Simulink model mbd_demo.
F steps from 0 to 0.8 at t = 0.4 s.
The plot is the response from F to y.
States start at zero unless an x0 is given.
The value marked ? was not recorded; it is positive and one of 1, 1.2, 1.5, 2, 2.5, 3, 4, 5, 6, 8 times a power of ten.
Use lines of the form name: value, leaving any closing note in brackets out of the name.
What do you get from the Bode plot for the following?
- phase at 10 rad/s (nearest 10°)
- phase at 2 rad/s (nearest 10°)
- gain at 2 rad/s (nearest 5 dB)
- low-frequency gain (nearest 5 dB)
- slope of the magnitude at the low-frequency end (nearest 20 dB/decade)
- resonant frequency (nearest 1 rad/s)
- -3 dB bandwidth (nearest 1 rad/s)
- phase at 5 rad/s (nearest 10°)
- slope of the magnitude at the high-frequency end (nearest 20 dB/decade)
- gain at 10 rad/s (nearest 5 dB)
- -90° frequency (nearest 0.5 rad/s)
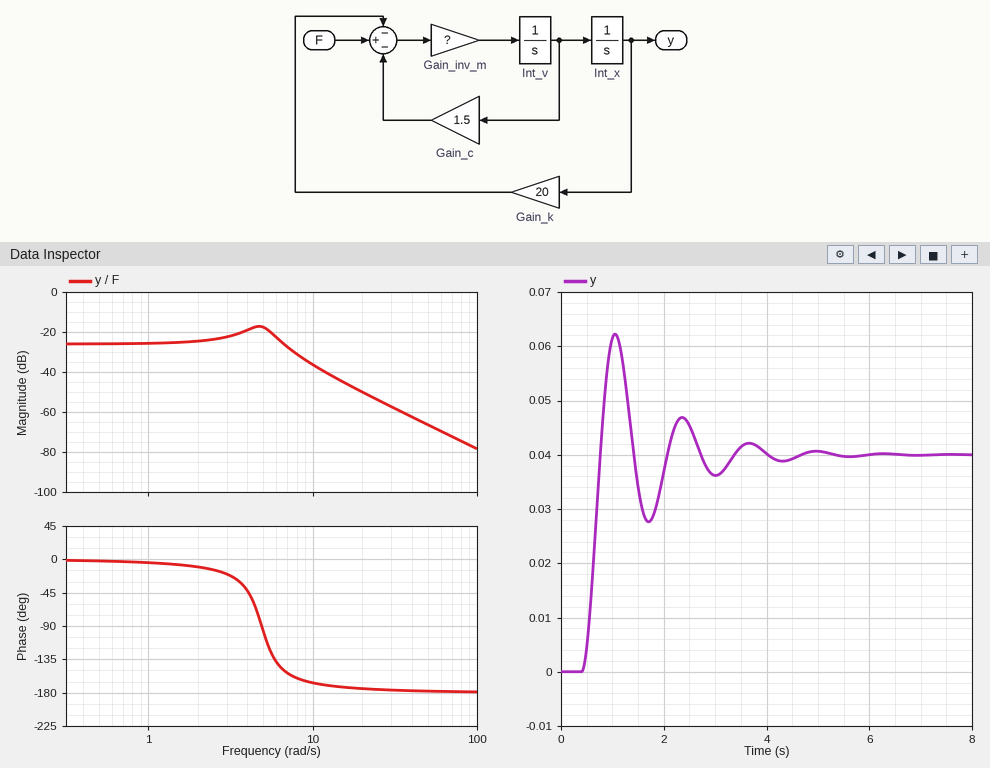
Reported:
phase at 10 rad/s: -170°
phase at 2 rad/s: -10°
gain at 2 rad/s: -25 dB
low-frequency gain: -25 dB
slope of the magnitude at the low-frequency end: 0 dB/decade
resonant frequency: 5 rad/s
-3 dB bandwidth: 7 rad/s
phase at 5 rad/s: -100°
slope of the magnitude at the high-frequency end: -40 dB/decade
gain at 10 rad/s: -35 dB
-90° frequency: 5.0 rad/s
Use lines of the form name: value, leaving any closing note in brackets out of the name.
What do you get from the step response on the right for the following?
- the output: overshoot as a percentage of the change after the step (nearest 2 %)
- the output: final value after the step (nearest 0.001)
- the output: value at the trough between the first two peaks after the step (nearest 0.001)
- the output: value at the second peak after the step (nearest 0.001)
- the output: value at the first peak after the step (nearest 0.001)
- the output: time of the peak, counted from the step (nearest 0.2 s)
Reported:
the output: overshoot as a percentage of the change after the step: 56 %
the output: final value after the step: 0.040
the output: value at the trough between the first two peaks after the step: 0.028
the output: value at the second peak after the step: 0.047
the output: value at the first peak after the step: 0.062
the output: time of the peak, counted from the step: 0.6 s
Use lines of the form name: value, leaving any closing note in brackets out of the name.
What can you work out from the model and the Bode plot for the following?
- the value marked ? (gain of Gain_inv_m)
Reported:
the value marked ?: 1.2
